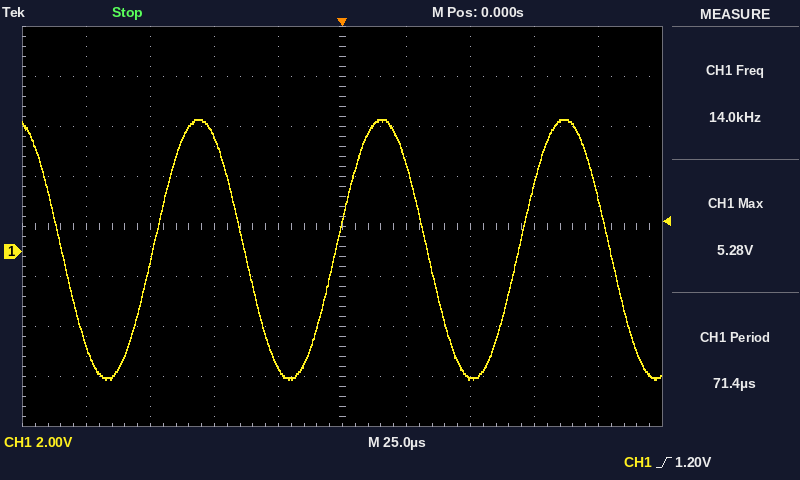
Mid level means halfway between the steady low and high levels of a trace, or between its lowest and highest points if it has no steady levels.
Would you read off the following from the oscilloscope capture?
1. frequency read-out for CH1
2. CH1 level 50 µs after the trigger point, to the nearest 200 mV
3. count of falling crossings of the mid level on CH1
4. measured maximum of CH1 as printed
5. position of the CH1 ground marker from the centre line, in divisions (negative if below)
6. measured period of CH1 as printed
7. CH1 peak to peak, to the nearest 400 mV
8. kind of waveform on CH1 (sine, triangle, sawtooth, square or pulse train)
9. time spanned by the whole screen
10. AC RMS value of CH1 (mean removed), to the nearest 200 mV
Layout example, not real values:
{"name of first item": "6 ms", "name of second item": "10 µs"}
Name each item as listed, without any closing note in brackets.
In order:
{"frequency read-out for CH1": "14.0 kHz", "CH1 level 50 µs after the trigger point, to the nearest 200 mV": "-5.0 V", "count of falling crossings of the mid level on CH1": "4", "measured maximum of CH1 as printed": "5.28 V", "position of the CH1 ground marker from the centre line, in divisions": "-0.5 div", "measured period of CH1 as printed": "71.4 µs", "CH1 peak to peak, to the nearest 400 mV": "10.4 V", "kind of waveform on CH1": "sine", "time spanned by the whole screen": "250 µs", "AC RMS value of CH1 (mean removed), to the nearest 200 mV": "3.6 V"}
